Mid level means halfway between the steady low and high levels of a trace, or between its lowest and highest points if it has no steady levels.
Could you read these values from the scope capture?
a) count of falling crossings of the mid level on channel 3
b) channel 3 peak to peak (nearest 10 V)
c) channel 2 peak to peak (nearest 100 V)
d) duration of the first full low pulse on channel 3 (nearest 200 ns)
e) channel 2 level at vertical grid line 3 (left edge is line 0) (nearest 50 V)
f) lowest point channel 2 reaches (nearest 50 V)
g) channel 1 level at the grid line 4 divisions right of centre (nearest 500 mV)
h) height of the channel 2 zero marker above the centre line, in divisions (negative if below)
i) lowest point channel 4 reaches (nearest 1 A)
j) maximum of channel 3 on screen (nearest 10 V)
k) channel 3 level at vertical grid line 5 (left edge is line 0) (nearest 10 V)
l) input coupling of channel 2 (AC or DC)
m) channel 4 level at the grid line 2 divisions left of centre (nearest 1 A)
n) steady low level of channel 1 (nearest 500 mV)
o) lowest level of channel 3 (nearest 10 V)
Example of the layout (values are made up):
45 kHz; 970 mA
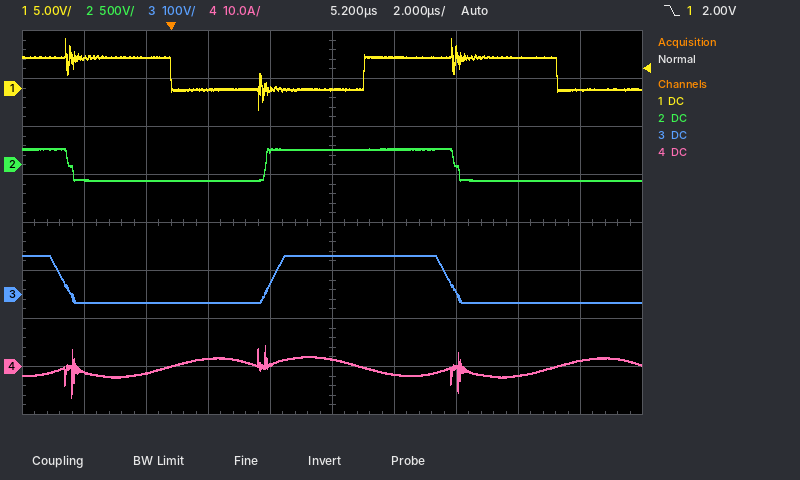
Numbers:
2; 100 V; 300 V; 6.8 µs; -150 V; -150 V; 0.0 V; +1.2 div; -6 A; 80 V; 80 V; DC; 2 A; 0.0 V; -20 V
